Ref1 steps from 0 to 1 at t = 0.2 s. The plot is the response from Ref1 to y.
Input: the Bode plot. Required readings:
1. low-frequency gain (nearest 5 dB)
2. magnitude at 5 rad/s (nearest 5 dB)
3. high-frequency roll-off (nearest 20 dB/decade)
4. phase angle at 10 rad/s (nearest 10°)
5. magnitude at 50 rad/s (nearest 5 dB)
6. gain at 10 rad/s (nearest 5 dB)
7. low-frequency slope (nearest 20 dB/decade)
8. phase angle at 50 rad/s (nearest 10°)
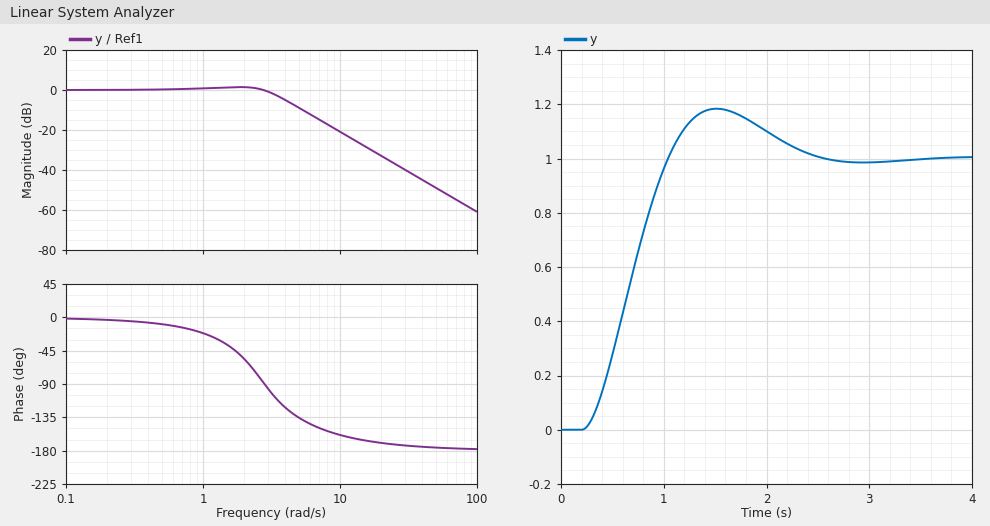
0 dB
-10 dB
-40 dB/decade
-160°
-50 dB
-20 dB
0 dB/decade
-180°
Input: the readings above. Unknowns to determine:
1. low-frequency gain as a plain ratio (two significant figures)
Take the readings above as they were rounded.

1.0
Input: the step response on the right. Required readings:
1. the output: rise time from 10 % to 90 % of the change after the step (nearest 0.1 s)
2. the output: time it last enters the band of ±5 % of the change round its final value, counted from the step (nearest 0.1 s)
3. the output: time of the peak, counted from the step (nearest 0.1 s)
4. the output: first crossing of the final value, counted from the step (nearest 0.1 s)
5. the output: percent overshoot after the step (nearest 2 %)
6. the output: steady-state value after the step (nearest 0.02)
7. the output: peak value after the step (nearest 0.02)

0.6 s
2.0 s
1.3 s
0.8 s
18 %
1.00
1.18
